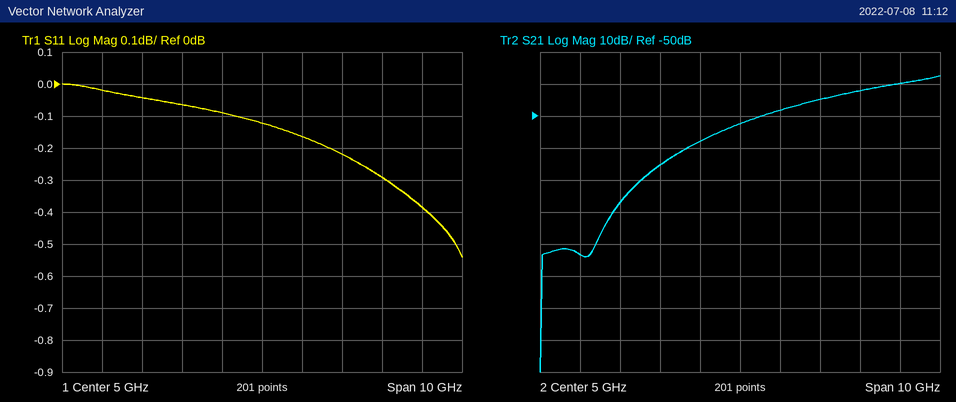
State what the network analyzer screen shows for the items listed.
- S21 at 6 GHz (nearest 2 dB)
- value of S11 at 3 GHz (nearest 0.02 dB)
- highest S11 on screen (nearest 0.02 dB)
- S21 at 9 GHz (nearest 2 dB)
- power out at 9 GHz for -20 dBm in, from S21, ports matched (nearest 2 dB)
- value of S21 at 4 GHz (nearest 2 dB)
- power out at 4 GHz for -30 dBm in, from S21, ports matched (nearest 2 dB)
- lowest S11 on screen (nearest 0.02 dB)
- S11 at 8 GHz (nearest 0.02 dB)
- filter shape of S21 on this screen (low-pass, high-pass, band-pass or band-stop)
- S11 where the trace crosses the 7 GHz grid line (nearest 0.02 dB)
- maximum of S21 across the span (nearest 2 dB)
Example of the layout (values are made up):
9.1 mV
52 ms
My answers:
-48 dB
-0.06 dB
0.00 dB
-40 dB
-60 dBm
-58 dB
-88 dBm
-0.54 dB
-0.30 dB
high-pass
-0.22 dB
-38 dB
